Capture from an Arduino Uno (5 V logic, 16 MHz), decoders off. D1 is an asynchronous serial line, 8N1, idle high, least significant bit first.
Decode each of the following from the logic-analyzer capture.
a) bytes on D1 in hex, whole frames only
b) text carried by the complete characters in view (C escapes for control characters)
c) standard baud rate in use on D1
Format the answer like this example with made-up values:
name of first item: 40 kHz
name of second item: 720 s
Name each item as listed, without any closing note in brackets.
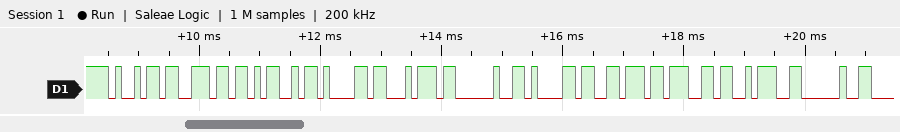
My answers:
bytes on D1 in hex, whole frames only: 0x69 0x6E 0x4D 0x61 0x74 0x20 0x61 0x76 0x67 0x3A 0x20
text carried by the complete characters in view: "inMat avg: "
standard baud rate in use on D1: 9600 baud
